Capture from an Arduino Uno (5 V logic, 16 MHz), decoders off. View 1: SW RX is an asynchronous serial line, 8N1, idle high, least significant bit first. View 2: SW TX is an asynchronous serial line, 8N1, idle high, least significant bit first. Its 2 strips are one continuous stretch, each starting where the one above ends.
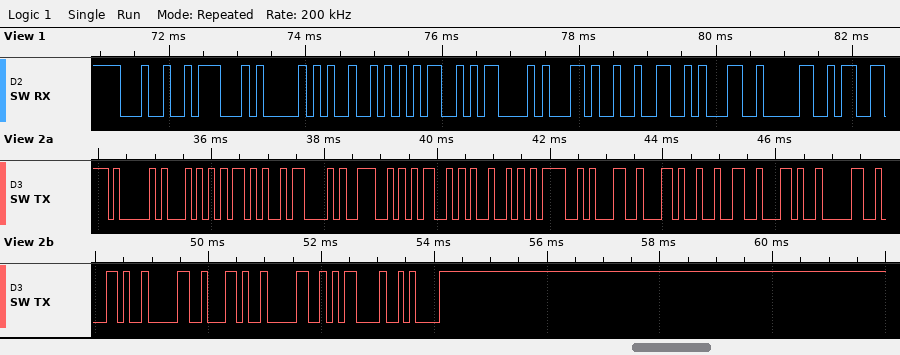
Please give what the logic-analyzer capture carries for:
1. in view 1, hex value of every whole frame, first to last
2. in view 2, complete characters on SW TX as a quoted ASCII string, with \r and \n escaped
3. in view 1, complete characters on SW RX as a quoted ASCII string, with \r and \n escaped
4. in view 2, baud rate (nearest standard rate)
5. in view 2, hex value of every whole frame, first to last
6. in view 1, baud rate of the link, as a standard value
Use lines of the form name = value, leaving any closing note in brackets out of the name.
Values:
in view 1, hex value of every whole frame, first to last = 24 47 50 52 4D 43 2C 32 31 30
in view 2, complete characters on SW TX as a quoted ASCII string, with \r and \n escaped = "AT+CNMI=1,2,0,0,0\r\n"
in view 1, complete characters on SW RX as a quoted ASCII string, with \r and \n escaped = "$GPRMC,210"
in view 2, baud rate = 9600 baud
in view 2, hex value of every whole frame, first to last = 41 54 2B 43 4E 4D 49 3D 31 2C 32 2C 30 2C 30 2C 30 0D 0A
in view 1, baud rate of the link, as a standard value = 9600 baud
